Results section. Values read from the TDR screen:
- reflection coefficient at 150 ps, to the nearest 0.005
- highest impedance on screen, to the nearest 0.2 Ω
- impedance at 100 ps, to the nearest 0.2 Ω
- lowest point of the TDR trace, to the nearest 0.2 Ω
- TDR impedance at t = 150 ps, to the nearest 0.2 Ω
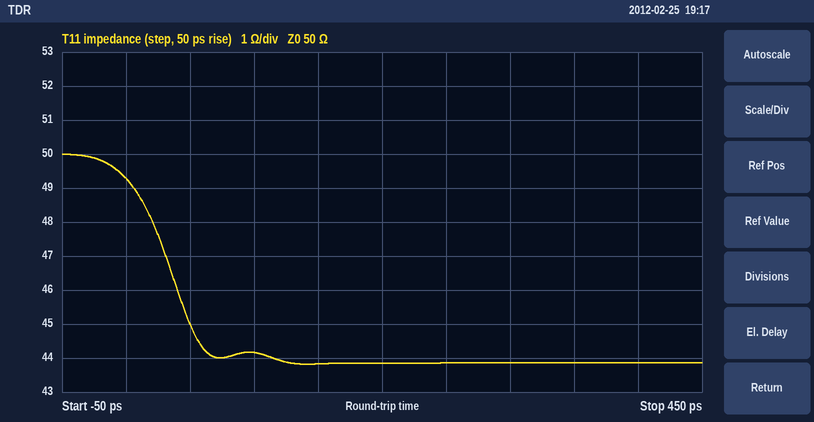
-0.065
50.0 Ω
44.2 Ω
43.8 Ω
43.8 Ω
